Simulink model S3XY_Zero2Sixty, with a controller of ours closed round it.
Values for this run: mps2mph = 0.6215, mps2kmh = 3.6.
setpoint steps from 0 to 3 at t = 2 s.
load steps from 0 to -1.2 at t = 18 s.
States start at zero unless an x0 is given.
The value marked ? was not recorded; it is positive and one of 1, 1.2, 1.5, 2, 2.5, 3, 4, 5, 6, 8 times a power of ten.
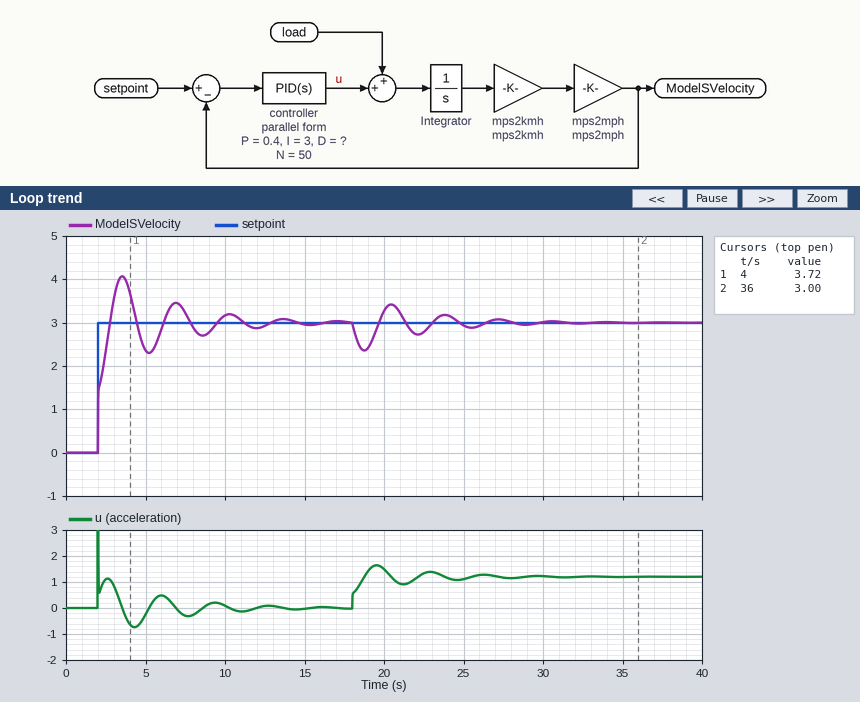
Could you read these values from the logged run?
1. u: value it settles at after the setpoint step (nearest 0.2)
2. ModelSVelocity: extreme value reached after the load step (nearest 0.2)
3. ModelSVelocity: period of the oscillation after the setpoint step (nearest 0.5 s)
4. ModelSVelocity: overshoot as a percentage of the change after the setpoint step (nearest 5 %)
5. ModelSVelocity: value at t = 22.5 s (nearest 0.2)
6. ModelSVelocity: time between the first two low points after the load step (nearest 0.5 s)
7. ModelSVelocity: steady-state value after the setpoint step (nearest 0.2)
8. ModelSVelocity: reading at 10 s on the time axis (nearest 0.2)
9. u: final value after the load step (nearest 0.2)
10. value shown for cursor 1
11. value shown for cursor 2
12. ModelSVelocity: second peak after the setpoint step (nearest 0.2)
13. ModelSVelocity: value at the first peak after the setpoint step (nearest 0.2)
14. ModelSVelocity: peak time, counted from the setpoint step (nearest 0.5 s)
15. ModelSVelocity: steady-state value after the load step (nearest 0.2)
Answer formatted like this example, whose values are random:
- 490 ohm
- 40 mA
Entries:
- 0.0
- 2.4
- 3.5 s
- 35 %
- 2.8
- 3.5 s
- 3.0
- 3.2
- 1.2
- 3.72
- 3.00
- 3.4
- 4.0
- 1.5 s
- 3.0
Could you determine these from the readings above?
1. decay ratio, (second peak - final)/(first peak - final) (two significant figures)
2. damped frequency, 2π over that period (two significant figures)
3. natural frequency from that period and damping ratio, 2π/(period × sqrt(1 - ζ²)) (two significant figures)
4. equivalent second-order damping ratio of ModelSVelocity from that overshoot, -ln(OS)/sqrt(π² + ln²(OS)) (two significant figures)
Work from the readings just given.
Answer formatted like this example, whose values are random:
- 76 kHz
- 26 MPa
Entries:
- 0.40
- 1.8 rad/s
- 1.9 rad/s
- 0.32
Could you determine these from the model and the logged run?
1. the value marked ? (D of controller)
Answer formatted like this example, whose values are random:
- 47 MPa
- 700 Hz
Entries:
- 0.4
